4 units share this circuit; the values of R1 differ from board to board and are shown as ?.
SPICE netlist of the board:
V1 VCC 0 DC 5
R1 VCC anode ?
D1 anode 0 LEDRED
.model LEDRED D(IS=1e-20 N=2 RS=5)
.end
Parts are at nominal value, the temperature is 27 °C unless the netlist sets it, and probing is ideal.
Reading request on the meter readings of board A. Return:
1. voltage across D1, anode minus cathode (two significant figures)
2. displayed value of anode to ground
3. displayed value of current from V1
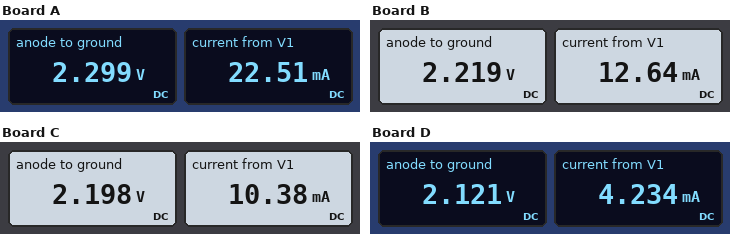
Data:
2.3 V
2.299 V
22.51 mA
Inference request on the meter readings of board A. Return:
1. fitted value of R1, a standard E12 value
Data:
120 Ω
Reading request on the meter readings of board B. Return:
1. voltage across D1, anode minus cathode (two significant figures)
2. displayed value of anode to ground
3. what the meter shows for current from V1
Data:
2.2 V
2.219 V
12.64 mA
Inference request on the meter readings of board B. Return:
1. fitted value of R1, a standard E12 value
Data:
220 Ω
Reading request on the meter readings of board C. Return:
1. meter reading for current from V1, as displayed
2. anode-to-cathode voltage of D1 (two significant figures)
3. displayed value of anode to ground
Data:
10.38 mA
2.2 V
2.198 V
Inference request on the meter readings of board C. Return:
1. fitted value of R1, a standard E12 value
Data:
270 Ω
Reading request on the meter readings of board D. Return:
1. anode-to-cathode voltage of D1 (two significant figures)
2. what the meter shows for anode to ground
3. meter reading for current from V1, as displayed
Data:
2.1 V
2.121 V
4.234 mA
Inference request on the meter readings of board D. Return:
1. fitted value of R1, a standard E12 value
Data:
680 Ω
